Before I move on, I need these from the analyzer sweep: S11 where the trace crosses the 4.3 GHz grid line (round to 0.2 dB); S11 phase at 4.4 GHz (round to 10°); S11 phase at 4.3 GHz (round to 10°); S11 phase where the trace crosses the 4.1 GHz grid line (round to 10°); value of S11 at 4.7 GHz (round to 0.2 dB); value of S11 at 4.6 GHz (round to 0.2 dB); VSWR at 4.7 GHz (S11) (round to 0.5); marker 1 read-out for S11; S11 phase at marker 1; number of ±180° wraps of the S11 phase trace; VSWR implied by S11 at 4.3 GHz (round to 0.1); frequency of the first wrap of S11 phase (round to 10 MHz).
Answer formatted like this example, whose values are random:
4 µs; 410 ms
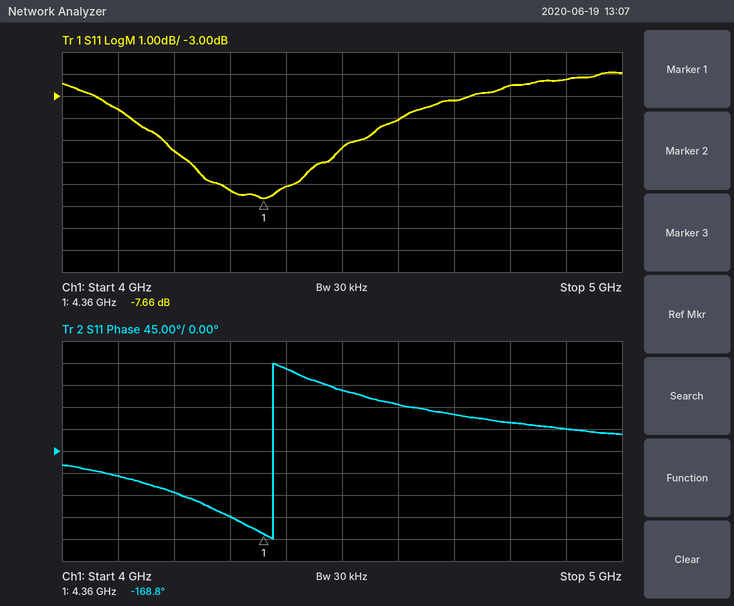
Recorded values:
-7.2 dB; 170°; -130°; -50°; -3.2 dB; -4.0 dB; 5.5; -7.66 dB; -168.8°; 1; 2.5; 4.38 GHz
